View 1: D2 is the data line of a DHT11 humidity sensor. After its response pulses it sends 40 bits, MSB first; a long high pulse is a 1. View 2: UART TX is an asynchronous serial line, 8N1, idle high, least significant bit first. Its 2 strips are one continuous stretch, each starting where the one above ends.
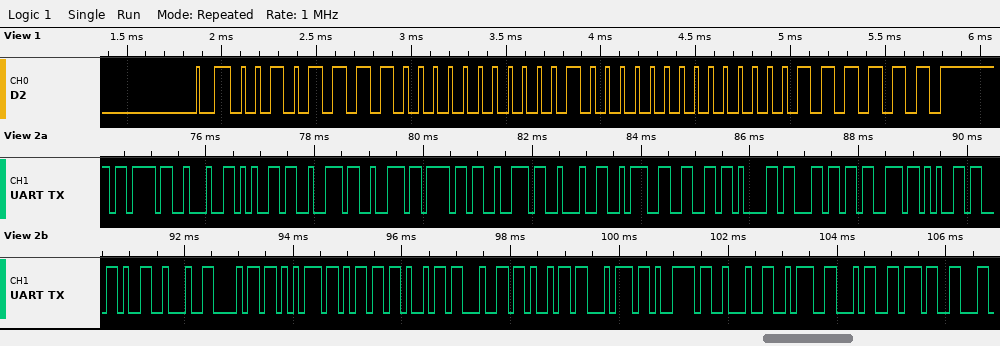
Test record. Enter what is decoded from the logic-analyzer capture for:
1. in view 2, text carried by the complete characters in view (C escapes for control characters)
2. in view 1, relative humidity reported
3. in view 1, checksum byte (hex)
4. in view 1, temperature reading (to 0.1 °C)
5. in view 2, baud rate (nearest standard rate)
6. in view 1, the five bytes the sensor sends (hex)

"{\"error\":false,\"humidity\":47"
47 %
0x3F
16.0 °C
9600 baud
2F 00 10 00 3F
